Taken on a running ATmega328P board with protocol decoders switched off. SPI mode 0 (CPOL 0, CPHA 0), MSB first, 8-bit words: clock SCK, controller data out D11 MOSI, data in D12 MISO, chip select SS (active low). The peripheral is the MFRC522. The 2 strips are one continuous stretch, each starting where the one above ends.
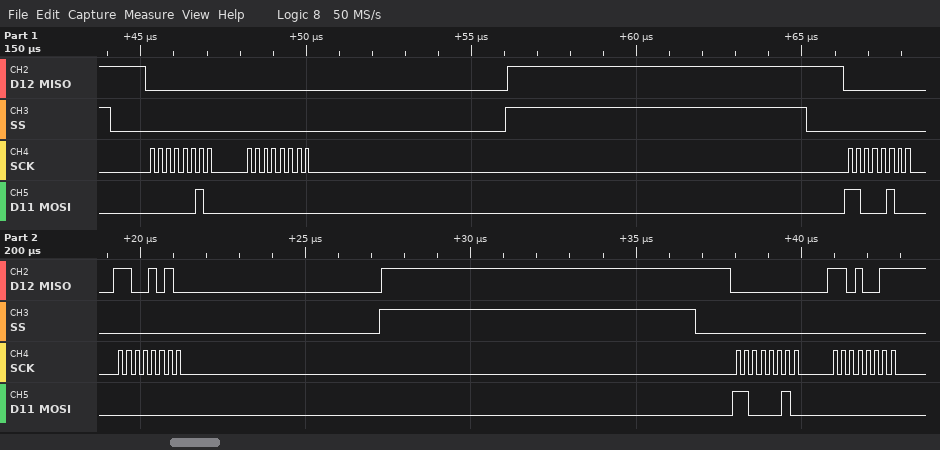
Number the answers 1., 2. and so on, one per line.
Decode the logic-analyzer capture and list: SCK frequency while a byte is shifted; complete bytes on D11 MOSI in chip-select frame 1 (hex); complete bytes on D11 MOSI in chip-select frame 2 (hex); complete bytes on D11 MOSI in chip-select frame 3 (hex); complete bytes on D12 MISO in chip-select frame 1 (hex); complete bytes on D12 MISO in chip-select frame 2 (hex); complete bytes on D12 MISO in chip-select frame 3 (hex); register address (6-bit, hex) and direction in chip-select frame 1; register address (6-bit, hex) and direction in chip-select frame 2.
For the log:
1. 4 MHz
2. 02 00
3. C4 00
4. C2 00
5. 00 00
6. 00 CA
7. 00 D3
8. 0x01 write
9. 0x22 read
